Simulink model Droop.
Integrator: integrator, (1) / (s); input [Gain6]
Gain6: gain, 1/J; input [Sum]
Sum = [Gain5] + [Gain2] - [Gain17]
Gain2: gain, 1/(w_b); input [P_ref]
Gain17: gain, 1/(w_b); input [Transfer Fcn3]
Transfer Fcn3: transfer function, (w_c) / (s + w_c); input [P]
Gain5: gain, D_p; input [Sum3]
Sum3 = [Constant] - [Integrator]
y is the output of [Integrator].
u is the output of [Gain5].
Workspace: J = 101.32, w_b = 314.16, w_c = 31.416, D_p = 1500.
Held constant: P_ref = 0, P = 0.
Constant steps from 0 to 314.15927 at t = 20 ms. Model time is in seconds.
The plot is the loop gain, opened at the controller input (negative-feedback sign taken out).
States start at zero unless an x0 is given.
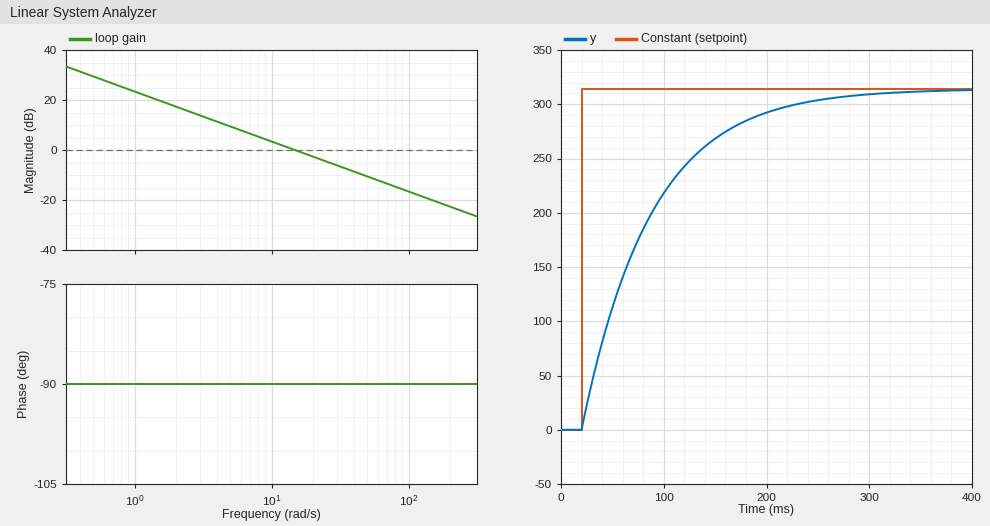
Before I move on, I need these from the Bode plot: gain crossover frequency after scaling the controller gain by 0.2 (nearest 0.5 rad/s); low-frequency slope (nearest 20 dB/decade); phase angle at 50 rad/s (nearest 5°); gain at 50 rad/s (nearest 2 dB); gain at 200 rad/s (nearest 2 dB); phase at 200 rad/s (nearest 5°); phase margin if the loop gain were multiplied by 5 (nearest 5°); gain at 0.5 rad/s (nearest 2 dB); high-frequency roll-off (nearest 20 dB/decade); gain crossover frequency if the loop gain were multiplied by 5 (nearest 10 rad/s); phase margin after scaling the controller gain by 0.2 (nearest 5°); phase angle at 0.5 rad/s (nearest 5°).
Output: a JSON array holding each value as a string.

["3.0 rad/s", "-20 dB/decade", "-90°", "-10 dB", "-22 dB", "-90°", "90°", "30 dB", "-20 dB/decade", "70 rad/s", "90°", "-90°"]
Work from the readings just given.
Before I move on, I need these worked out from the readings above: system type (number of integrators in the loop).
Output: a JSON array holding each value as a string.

["1"]
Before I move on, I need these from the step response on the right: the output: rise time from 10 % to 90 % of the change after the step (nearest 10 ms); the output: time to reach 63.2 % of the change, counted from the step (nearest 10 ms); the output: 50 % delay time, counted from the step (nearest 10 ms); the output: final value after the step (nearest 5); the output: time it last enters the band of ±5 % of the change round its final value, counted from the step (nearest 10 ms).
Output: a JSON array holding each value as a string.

["150 ms", "70 ms", "50 ms", "315", "200 ms"]
